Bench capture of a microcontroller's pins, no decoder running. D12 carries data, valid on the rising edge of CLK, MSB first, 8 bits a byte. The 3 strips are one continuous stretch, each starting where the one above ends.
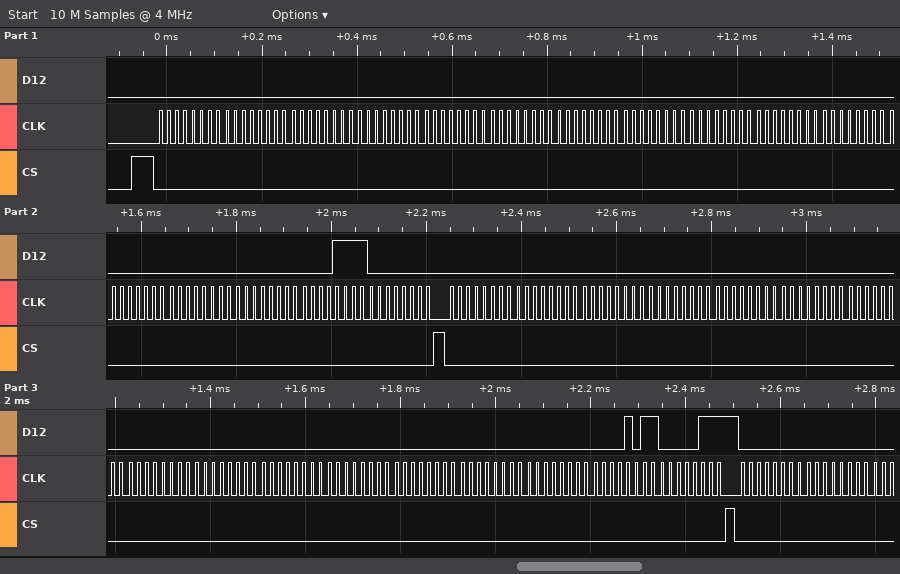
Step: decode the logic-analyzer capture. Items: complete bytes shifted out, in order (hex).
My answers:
00 00 00 00 00 00 00 00 00 00 00 00 00 00 0F 00 00 00 00 00 00 00 00 00 00 00 00 00 00 00 0B 07 00 00
